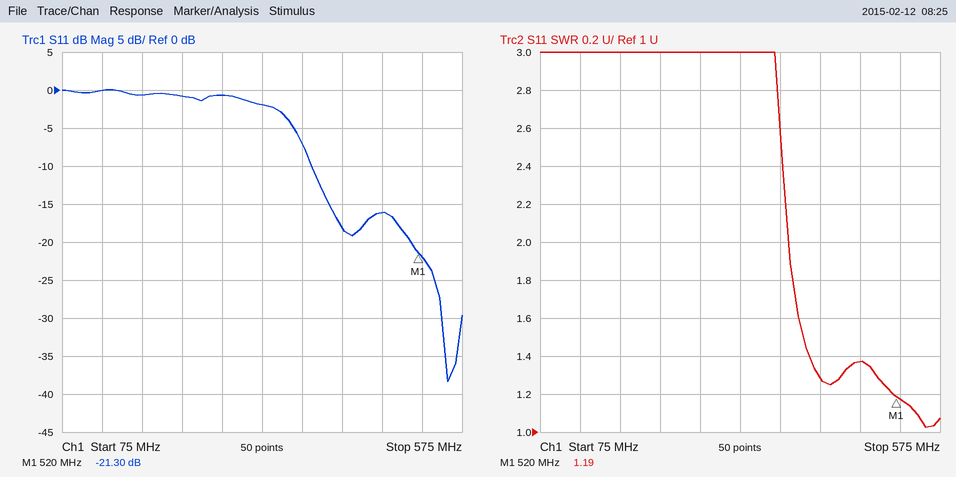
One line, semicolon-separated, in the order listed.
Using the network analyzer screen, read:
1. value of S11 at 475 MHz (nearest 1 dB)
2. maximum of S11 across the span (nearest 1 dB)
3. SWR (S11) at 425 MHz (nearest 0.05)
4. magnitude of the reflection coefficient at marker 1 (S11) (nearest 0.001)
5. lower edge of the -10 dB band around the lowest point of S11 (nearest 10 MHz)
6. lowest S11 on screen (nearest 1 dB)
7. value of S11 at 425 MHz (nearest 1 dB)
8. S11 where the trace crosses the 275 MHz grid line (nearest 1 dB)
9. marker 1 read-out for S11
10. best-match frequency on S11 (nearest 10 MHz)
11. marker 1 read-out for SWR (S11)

-16 dB; 0 dB; 1.30; 0.086; 390 MHz; -38 dB; -18 dB; -1 dB; -21.30 dB; 560 MHz; 1.19
